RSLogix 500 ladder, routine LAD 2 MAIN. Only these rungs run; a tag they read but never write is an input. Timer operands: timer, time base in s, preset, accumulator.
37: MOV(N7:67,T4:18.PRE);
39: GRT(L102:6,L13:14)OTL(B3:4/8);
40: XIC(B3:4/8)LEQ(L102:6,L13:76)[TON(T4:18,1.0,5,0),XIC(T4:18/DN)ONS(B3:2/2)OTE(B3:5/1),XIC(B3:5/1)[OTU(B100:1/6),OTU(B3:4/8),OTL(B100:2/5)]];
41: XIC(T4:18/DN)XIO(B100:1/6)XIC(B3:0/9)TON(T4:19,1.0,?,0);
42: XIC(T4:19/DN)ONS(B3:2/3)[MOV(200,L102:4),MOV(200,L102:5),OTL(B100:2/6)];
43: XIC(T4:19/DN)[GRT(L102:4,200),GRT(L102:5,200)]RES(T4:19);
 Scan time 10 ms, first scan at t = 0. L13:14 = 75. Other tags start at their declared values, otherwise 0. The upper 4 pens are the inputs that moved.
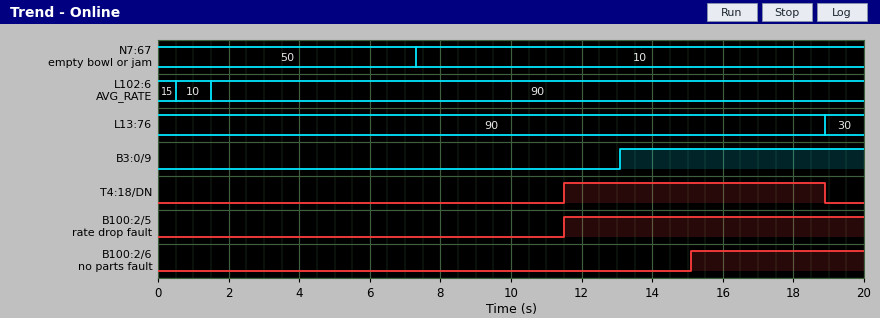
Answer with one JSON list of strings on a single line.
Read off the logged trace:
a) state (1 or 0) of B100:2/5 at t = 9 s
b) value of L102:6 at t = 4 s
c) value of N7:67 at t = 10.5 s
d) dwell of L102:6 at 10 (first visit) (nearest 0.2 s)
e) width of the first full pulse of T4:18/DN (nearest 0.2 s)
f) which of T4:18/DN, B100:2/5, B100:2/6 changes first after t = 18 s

["0", "90", "10", "1.0 s", "7.4 s", "T4:18/DN"]
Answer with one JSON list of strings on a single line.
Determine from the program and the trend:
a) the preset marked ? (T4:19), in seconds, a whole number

["2 s"]
